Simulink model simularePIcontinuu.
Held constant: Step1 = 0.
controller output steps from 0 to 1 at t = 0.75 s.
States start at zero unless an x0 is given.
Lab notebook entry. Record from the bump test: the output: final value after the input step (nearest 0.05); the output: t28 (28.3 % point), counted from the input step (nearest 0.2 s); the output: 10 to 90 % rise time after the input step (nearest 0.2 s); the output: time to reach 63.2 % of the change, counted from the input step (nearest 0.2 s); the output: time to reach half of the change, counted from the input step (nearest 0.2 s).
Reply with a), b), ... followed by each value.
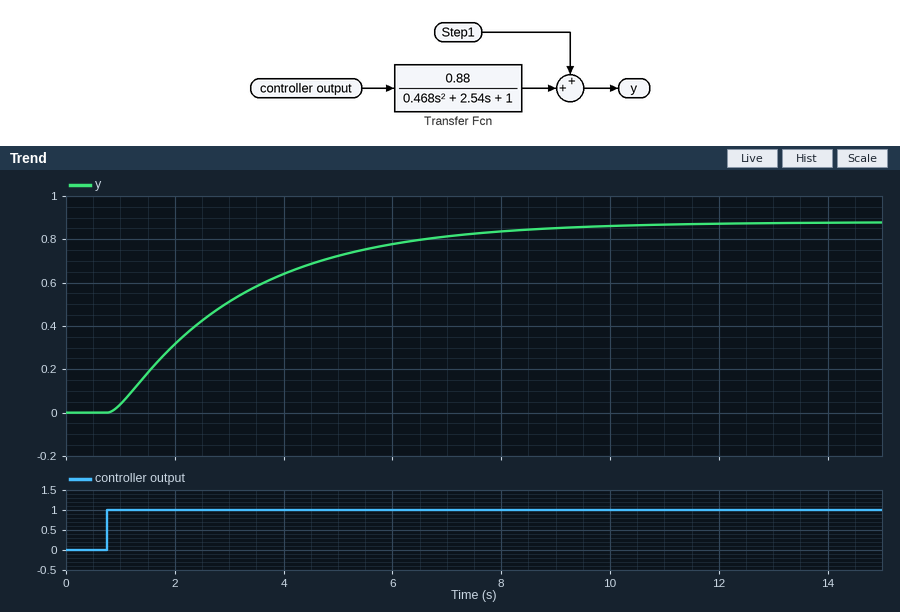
a) 0.90
b) 1.0 s
c) 5.2 s
d) 2.6 s
e) 1.8 s
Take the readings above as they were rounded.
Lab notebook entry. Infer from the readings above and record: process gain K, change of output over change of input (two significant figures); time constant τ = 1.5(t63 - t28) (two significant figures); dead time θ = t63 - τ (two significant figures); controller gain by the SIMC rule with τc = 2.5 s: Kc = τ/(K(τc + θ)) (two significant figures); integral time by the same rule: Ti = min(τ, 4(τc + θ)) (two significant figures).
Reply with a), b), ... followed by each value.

a) 0.90
b) 2.4 s
c) 0.20 s
d) 0.99
e) 2.4 s
